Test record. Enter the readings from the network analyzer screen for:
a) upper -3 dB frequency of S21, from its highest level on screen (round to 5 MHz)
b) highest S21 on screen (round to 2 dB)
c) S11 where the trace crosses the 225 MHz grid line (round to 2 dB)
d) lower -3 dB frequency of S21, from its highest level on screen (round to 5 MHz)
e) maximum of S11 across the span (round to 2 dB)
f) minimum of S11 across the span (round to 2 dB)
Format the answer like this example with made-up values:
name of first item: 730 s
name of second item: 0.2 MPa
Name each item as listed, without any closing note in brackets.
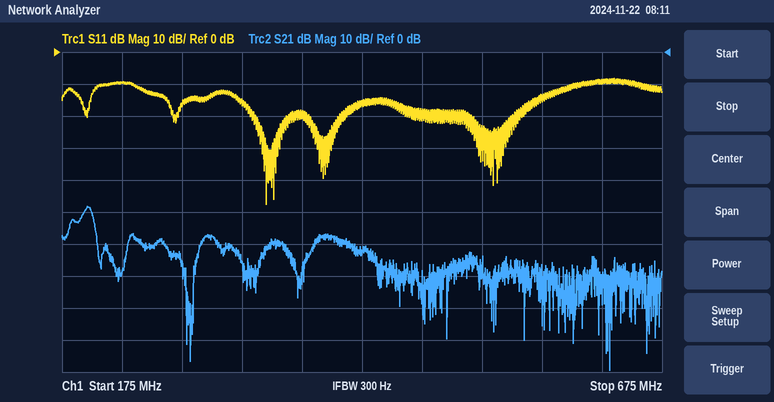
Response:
upper -3 dB frequency of S21, from its highest level on screen: 200 MHz
highest S21 on screen: -48 dB
S11 where the trace crosses the 225 MHz grid line: -10 dB
lower -3 dB frequency of S21, from its highest level on screen: 190 MHz
maximum of S11 across the span: -8 dB
minimum of S11 across the span: -48 dB
